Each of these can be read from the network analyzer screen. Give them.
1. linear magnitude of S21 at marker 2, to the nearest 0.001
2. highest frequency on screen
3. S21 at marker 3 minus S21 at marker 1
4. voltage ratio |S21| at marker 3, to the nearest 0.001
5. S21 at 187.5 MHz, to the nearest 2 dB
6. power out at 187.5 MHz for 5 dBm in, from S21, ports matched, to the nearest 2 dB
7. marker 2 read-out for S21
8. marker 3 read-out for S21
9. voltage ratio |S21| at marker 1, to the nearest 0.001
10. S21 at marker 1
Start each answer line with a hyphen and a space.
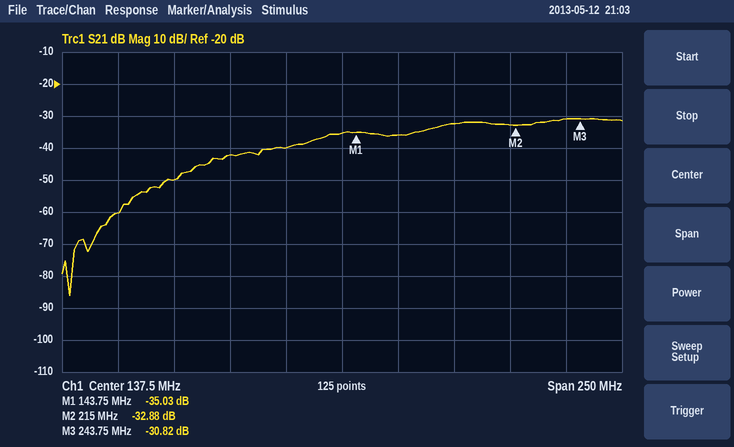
- 0.023
- 262.5 MHz
- 4.21 dB
- 0.029
- -32 dB
- -28 dBm
- -32.88 dB
- -30.82 dB
- 0.018
- -35.03 dB
